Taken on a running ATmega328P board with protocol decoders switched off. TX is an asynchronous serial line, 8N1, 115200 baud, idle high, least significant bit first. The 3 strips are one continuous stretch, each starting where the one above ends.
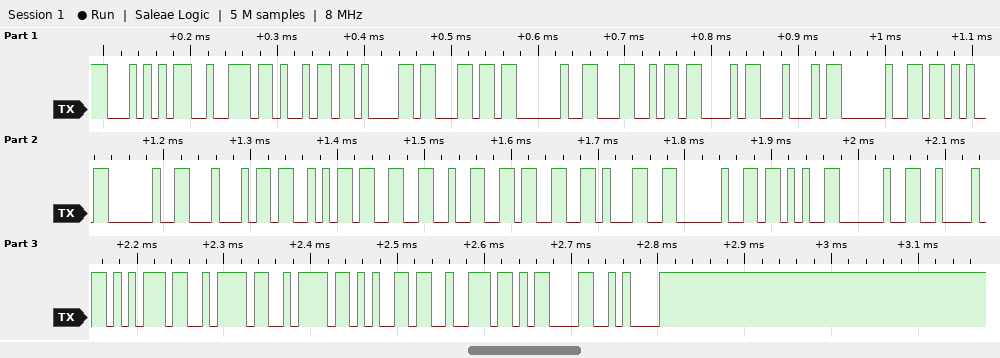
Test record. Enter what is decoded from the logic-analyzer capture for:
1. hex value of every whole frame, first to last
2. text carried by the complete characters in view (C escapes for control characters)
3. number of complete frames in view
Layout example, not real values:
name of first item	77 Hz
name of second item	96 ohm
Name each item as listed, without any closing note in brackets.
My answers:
hex value of every whole frame, first to last	54 72 69 61 6C 20 4C 43 44 20 2B 20 44 53 33 32 33 31 20 2B 20 42 75 7A 7A 65 72 0D 0A
text carried by the complete characters in view	"Trial LCD + DS3231 + Buzzer\r\n"
number of complete frames in view	29
